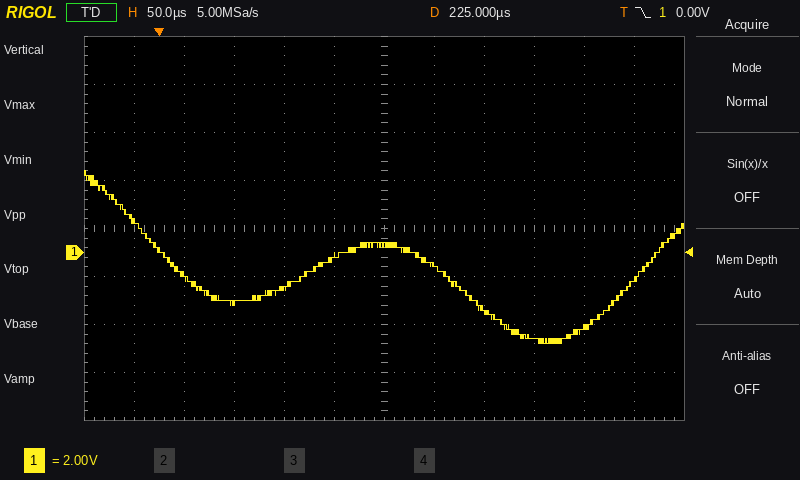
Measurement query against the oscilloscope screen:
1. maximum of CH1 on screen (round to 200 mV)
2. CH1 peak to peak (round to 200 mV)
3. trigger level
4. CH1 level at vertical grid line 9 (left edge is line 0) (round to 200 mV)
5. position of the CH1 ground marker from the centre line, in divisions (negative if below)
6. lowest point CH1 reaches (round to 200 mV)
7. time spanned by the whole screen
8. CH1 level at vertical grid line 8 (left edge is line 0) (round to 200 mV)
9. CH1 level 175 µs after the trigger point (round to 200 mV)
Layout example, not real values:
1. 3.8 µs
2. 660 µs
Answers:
1. 3.4 V
2. 7.2 V
3. 0.00 V
4. -3.6 V
5. -0.5 div
6. -3.8 V
7. 600 µs
8. -2.4 V
9. -200 mV
